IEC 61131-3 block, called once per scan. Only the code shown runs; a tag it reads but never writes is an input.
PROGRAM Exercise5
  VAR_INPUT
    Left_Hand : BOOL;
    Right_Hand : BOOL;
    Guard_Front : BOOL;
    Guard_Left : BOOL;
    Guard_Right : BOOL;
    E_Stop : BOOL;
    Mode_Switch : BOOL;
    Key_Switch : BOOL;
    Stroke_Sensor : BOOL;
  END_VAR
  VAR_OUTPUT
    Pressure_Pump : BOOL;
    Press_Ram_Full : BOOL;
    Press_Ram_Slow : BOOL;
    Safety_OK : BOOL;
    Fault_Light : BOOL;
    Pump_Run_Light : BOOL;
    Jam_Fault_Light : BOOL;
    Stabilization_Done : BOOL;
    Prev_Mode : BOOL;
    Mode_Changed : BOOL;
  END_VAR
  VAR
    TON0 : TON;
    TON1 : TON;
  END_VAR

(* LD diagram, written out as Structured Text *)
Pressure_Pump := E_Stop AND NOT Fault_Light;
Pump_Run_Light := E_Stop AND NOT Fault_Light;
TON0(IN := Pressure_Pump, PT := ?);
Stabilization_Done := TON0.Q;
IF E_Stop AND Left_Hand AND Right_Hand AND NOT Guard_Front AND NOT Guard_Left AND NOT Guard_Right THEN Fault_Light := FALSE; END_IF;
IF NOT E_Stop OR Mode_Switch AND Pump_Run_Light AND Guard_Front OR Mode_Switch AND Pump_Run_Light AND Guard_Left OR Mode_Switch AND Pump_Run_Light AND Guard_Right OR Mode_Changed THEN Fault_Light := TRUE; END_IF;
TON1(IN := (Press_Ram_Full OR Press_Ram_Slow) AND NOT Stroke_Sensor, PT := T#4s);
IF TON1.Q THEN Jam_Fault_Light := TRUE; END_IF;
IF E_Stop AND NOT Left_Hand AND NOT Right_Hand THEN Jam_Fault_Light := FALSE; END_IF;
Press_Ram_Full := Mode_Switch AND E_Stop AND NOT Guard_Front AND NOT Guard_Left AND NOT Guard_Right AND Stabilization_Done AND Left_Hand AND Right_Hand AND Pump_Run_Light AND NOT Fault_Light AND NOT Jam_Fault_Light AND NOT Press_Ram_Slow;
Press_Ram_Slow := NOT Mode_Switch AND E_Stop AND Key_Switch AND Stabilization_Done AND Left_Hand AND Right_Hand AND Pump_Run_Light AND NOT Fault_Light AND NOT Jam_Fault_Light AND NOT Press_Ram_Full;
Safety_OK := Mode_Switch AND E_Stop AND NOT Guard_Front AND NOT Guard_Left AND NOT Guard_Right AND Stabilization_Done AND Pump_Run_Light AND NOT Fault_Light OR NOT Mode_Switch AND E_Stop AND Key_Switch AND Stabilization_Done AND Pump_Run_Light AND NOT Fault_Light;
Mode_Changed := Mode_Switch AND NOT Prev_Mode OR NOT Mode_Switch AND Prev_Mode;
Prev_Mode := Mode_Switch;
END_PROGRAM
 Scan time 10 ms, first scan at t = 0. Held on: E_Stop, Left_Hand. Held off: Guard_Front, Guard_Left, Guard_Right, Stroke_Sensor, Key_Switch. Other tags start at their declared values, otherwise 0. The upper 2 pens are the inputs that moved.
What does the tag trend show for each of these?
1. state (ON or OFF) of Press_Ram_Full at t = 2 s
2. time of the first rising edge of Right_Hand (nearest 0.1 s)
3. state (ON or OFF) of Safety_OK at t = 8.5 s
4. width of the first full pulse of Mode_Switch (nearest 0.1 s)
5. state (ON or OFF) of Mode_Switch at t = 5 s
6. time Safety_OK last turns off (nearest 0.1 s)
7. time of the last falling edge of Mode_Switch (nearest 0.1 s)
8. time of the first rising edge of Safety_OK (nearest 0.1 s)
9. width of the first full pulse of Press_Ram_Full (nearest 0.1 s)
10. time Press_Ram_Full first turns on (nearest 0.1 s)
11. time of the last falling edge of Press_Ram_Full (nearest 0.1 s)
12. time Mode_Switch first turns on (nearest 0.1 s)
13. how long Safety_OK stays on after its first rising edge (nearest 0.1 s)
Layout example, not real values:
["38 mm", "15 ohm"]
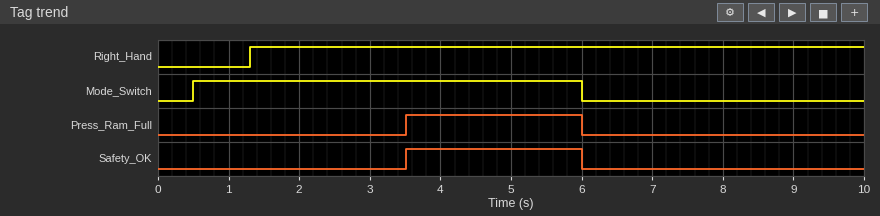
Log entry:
["OFF", "1.3 s", "OFF", "5.5 s", "ON", "6.0 s", "6.0 s", "3.5 s", "2.5 s", "3.5 s", "6.0 s", "0.5 s", "2.5 s"]
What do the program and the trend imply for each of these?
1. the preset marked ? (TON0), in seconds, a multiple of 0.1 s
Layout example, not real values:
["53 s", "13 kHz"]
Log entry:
["2.2 s"]
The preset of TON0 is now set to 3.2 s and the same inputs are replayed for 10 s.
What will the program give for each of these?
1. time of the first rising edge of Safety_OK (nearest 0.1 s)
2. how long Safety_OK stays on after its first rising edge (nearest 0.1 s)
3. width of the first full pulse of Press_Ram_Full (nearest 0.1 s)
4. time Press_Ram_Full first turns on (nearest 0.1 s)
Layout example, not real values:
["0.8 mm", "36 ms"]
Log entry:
["4.5 s", "1.5 s", "1.5 s", "4.5 s"]
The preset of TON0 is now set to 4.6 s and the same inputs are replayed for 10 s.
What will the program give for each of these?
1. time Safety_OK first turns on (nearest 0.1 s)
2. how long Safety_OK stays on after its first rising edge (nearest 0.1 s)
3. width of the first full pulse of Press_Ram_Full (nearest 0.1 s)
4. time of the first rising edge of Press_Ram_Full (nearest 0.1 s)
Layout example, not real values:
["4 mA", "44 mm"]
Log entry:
["5.9 s", "0.1 s", "0.1 s", "5.9 s"]
